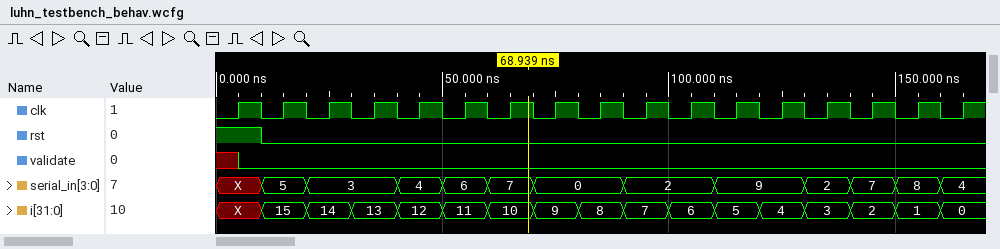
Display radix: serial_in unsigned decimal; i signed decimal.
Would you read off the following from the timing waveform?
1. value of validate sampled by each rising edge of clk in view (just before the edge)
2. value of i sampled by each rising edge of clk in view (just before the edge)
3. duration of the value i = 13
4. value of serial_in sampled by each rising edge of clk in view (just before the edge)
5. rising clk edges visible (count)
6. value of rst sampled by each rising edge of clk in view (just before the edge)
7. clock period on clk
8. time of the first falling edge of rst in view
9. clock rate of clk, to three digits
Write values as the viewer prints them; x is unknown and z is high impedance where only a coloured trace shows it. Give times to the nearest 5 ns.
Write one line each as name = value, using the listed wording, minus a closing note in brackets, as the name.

value of validate sampled by each rising edge of clk in view = x 0 0 0 0 0 0 0 0 0 0 0 0 0 0 0 0
value of i sampled by each rising edge of clk in view = X, 15, 14, 13, 12, 11, 10, 9, 8, 7, 6, 5, 4, 3, 2, 1, 0
duration of the value i = 13 = 10 ns
value of serial_in sampled by each rising edge of clk in view = X, 5, 3, 3, 4, 6, 7, 0, 0, 2, 2, 9, 9, 2, 7, 8, 4
rising clk edges visible = 17
value of rst sampled by each rising edge of clk in view = 1 0 0 0 0 0 0 0 0 0 0 0 0 0 0 0 0
clock period on clk = 10 ns
time of the first falling edge of rst in view = 10 ns
clock rate of clk, to three digits = 100 MHz
